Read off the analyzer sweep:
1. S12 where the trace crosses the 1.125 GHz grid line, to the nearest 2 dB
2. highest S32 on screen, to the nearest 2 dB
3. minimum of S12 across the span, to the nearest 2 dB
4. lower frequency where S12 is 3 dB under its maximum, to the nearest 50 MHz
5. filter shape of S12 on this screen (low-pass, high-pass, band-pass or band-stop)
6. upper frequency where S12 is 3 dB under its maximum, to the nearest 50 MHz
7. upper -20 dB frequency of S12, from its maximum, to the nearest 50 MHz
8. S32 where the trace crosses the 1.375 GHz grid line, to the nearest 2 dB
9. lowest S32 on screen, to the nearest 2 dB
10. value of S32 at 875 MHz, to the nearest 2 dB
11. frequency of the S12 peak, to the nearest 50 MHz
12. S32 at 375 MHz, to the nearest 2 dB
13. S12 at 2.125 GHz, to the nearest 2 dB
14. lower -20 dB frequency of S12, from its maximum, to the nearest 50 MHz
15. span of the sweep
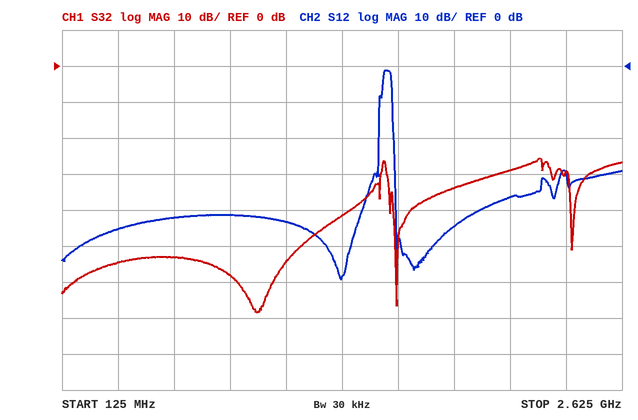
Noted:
-44 dB
-26 dB
-60 dB
1.55 GHz
band-pass
1.60 GHz
1.60 GHz
-42 dB
-68 dB
-58 dB
1.55 GHz
-54 dB
-36 dB
1.55 GHz
2.5 GHz
